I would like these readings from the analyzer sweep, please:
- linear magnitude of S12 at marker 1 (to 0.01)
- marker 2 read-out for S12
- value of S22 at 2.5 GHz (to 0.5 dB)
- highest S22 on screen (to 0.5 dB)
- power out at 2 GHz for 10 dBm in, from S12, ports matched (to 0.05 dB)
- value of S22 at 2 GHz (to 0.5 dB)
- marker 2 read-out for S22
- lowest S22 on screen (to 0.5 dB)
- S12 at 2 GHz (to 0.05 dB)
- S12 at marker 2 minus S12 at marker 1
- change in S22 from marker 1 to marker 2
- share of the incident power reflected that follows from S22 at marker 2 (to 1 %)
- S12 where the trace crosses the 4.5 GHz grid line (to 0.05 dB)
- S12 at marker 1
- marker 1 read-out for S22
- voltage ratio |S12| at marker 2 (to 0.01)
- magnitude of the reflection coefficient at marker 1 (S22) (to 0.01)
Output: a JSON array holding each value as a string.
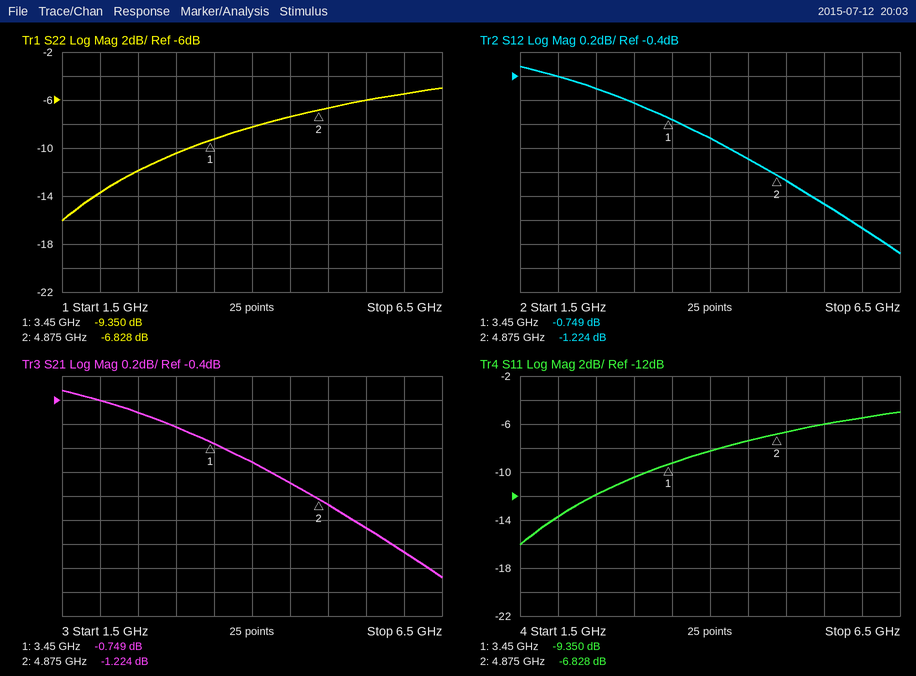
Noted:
["0.92", "-1.224 dB", "-12.0 dB", "-5.0 dB", "9.60 dBm", "-13.5 dB", "-6.828 dB", "-16.0 dB", "-0.40 dB", "-0.475 dB", "2.522 dB", "21 %", "-1.10 dB", "-0.749 dB", "-9.350 dB", "0.87", "0.34"]
